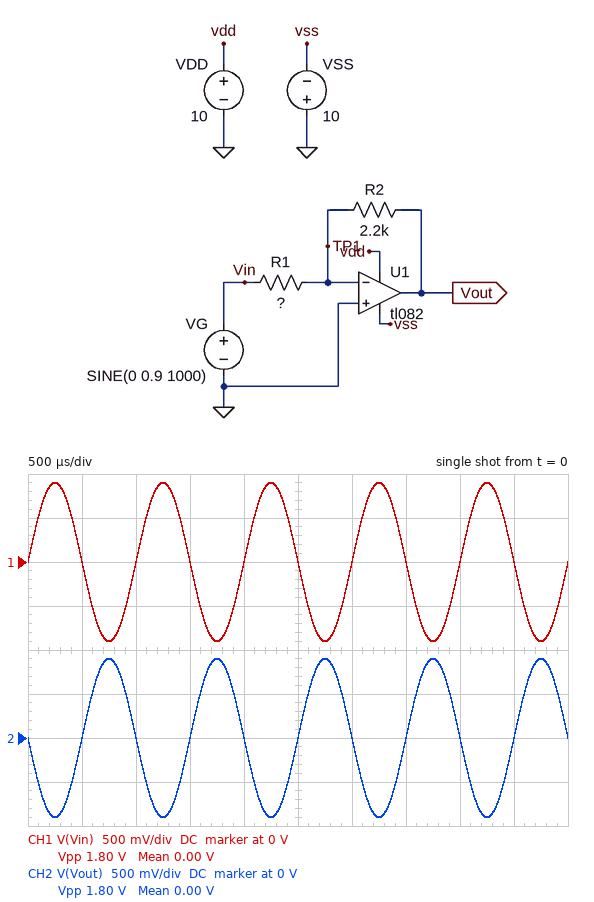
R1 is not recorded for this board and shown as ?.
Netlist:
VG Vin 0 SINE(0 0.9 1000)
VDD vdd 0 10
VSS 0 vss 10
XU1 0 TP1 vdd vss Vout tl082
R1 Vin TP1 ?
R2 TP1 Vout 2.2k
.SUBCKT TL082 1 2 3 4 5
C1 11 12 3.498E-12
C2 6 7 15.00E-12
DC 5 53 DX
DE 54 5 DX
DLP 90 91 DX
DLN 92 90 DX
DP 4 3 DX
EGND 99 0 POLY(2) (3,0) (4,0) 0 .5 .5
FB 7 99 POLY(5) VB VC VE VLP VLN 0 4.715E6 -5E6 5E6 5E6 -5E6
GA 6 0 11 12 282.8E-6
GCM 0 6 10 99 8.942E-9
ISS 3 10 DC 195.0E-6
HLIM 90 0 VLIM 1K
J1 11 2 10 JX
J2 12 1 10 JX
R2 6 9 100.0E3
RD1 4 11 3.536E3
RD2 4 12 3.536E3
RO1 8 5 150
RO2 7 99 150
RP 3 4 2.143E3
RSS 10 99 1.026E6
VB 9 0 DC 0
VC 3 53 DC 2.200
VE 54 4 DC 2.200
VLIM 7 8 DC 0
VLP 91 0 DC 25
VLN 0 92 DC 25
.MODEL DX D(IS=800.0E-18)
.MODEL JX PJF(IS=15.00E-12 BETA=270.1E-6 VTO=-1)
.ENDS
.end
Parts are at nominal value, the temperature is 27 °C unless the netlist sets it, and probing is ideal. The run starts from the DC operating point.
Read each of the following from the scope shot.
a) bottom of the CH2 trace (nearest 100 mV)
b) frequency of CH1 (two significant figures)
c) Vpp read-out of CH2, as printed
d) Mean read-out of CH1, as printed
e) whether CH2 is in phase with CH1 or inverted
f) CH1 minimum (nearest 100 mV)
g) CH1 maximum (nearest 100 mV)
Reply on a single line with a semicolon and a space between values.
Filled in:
-900 mV; 1.0 kHz; 1.80 V; 0.00 V; inverted; -900 mV; 900 mV
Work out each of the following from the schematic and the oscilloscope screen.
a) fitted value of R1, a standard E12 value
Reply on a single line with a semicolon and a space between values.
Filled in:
2.2 kΩ
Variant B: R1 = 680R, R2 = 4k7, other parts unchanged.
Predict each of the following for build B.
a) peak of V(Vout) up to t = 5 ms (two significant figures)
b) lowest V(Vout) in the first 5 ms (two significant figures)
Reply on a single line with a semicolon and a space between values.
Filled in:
6.2 V; -6.2 V
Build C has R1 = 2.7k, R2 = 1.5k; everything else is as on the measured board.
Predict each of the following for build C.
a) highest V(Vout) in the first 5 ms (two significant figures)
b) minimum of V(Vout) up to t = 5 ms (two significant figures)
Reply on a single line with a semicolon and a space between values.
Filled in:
500 mV; -500 mV
